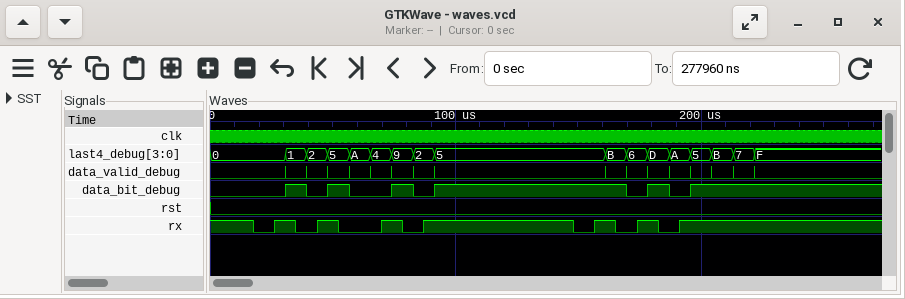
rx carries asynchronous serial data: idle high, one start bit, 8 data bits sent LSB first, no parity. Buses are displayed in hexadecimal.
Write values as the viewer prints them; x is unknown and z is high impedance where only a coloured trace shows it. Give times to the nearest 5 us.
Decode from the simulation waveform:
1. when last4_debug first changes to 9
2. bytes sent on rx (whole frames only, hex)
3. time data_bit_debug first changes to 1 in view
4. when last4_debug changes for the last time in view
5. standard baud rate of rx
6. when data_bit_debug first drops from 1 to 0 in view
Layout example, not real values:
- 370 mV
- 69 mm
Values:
- 75 us
- A5, F5
- 30 us
- 220 us
- 115200 baud
- 40 us
